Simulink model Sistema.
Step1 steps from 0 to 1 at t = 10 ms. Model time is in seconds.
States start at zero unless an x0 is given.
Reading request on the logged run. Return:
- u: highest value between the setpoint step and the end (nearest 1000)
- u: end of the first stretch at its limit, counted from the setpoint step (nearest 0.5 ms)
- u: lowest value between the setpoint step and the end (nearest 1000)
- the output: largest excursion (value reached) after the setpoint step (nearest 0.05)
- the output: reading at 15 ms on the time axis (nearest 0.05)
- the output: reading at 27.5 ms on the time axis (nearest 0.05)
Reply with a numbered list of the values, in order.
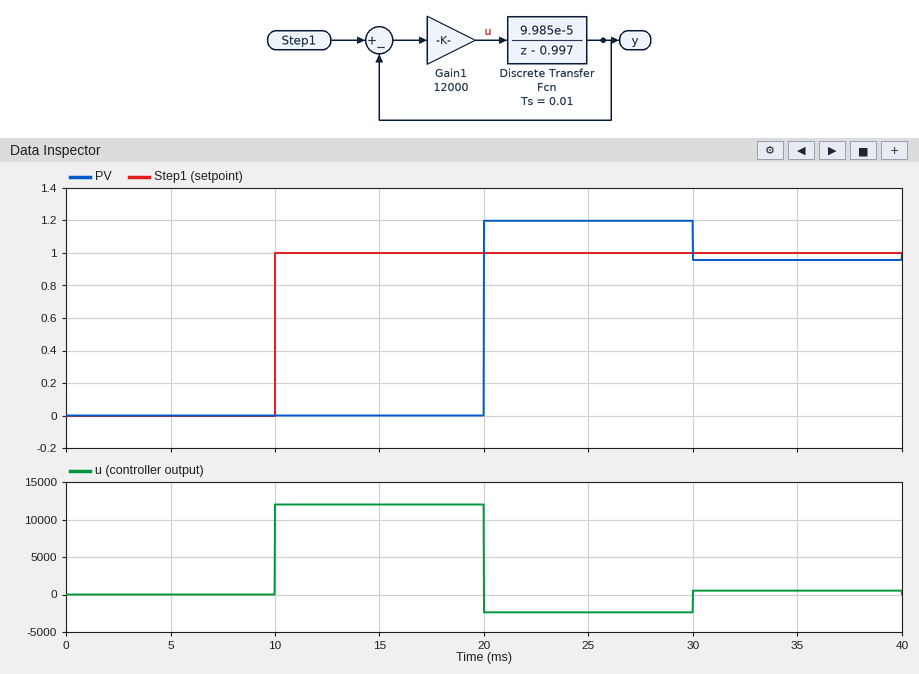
1. 12000
2. 10.0 ms
3. -2000
4. 1.20
5. 0.00
6. 1.20
